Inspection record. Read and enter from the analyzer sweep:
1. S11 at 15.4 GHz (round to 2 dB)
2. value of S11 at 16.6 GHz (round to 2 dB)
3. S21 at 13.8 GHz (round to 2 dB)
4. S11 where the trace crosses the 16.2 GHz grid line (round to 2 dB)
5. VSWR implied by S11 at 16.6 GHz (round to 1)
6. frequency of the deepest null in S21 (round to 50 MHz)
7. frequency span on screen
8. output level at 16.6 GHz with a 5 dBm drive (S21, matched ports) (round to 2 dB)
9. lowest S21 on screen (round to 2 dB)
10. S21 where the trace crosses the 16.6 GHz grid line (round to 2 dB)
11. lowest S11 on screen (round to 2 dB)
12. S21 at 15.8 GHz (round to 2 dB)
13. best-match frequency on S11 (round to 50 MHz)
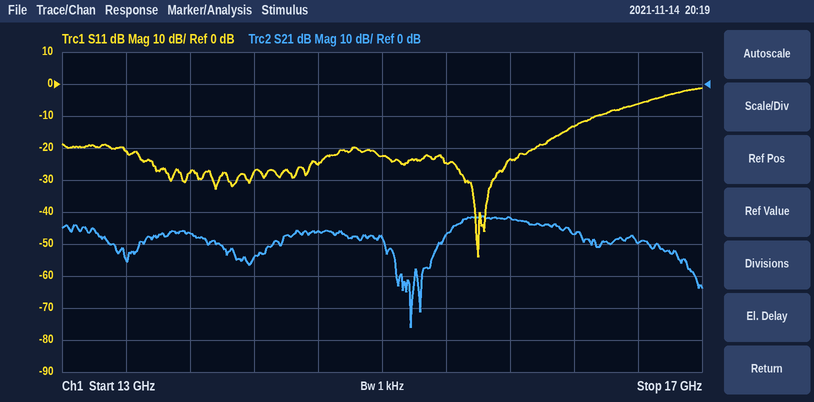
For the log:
-24 dB
-6 dB
-46 dB
-14 dB
3
15.20 GHz
4 GHz
-44 dBm
-76 dB
-50 dB
-54 dB
-42 dB
15.60 GHz
